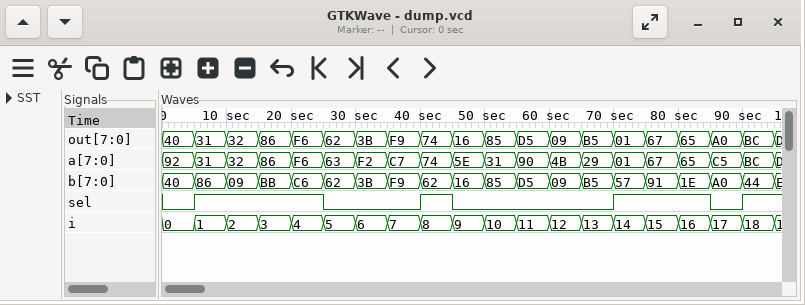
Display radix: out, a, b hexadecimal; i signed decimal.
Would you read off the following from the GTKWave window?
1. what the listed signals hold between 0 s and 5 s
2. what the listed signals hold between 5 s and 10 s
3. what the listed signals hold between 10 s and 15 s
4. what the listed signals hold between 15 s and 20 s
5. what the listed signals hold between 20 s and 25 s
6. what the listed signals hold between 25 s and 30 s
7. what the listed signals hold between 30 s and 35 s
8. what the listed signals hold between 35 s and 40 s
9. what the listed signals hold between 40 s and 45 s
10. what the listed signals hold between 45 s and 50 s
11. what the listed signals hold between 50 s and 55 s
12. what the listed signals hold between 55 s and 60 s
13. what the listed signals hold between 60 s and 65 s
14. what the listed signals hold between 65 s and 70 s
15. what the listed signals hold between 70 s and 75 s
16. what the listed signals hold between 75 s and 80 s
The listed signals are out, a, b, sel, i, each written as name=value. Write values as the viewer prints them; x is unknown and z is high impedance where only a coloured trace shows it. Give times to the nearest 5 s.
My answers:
out=40, a=92, b=40, sel=0, i=0
out=31, a=31, b=86, sel=1, i=1
out=32, a=32, b=09, sel=1, i=2
out=86, a=86, b=BB, sel=1, i=3
out=F6, a=F6, b=C6, sel=1, i=4
out=62, a=63, b=62, sel=0, i=5
out=3B, a=F2, b=3B, sel=0, i=6
out=F9, a=C7, b=F9, sel=0, i=7
out=74, a=74, b=62, sel=1, i=8
out=16, a=5E, b=16, sel=0, i=9
out=85, a=31, b=85, sel=0, i=10
out=D5, a=90, b=D5, sel=0, i=11
out=09, a=4B, b=09, sel=0, i=12
out=B5, a=29, b=B5, sel=0, i=13
out=01, a=01, b=57, sel=1, i=14
out=67, a=67, b=91, sel=1, i=15
